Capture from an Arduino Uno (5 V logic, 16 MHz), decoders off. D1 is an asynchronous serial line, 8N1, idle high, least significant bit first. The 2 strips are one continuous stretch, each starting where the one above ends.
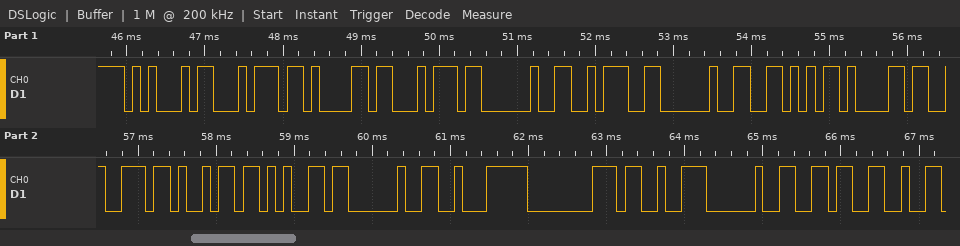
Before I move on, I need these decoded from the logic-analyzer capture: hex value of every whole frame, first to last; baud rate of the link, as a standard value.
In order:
45 74 61 74 20 3A 20 56 61 72 69 65 20 E2 80 93 20 36
9600 baud
